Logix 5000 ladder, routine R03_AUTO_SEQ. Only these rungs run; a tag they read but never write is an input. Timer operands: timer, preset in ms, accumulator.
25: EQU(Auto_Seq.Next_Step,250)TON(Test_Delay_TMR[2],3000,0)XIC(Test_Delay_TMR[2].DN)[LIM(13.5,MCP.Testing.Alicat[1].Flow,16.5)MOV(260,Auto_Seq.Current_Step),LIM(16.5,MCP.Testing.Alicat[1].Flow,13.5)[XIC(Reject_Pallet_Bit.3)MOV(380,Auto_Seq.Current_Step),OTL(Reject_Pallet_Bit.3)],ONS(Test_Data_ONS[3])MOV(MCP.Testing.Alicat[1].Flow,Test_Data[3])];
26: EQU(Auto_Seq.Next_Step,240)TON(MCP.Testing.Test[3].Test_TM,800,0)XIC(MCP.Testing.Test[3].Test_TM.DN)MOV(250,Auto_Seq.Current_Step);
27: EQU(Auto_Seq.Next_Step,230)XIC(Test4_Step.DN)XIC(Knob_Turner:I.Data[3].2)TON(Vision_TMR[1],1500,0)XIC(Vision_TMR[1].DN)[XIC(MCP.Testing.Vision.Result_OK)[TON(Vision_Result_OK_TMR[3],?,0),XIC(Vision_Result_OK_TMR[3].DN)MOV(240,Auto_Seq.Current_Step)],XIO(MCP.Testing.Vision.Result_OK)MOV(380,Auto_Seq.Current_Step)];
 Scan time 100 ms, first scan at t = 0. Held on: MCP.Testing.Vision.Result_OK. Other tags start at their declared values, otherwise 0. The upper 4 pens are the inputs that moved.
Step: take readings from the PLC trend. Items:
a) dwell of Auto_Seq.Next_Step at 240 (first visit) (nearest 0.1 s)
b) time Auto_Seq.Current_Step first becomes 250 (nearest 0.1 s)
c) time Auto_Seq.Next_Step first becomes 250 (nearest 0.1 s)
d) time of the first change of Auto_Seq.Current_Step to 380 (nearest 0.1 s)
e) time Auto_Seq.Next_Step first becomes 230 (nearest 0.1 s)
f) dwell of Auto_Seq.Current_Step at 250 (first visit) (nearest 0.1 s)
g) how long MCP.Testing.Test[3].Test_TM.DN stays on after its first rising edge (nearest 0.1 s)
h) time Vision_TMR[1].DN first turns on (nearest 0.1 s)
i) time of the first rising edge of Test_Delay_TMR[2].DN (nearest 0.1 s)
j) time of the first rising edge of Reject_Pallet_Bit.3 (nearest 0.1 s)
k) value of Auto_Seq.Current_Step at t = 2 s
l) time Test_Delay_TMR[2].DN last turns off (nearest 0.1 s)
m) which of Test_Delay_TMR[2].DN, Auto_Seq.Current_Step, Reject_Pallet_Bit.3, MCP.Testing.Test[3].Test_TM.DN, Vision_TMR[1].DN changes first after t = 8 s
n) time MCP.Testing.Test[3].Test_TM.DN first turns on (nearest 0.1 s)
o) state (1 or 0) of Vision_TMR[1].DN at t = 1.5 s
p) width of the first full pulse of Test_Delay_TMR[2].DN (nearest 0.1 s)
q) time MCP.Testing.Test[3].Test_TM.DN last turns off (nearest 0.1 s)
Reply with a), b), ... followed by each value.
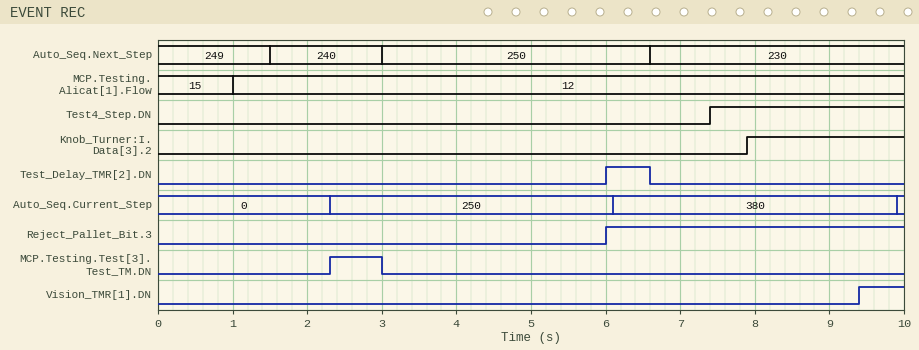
a) 1.5 s
b) 2.3 s
c) 3.0 s
d) 6.1 s
e) 6.6 s
f) 3.8 s
g) 0.7 s
h) 9.4 s
i) 6.0 s
j) 6.0 s
k) 0
l) 6.6 s
m) Vision_TMR[1].DN
n) 2.3 s
o) 0
p) 0.6 s
q) 3.0 s
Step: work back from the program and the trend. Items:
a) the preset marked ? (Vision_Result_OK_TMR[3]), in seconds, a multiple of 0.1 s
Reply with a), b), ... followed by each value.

a) 0.5 s
